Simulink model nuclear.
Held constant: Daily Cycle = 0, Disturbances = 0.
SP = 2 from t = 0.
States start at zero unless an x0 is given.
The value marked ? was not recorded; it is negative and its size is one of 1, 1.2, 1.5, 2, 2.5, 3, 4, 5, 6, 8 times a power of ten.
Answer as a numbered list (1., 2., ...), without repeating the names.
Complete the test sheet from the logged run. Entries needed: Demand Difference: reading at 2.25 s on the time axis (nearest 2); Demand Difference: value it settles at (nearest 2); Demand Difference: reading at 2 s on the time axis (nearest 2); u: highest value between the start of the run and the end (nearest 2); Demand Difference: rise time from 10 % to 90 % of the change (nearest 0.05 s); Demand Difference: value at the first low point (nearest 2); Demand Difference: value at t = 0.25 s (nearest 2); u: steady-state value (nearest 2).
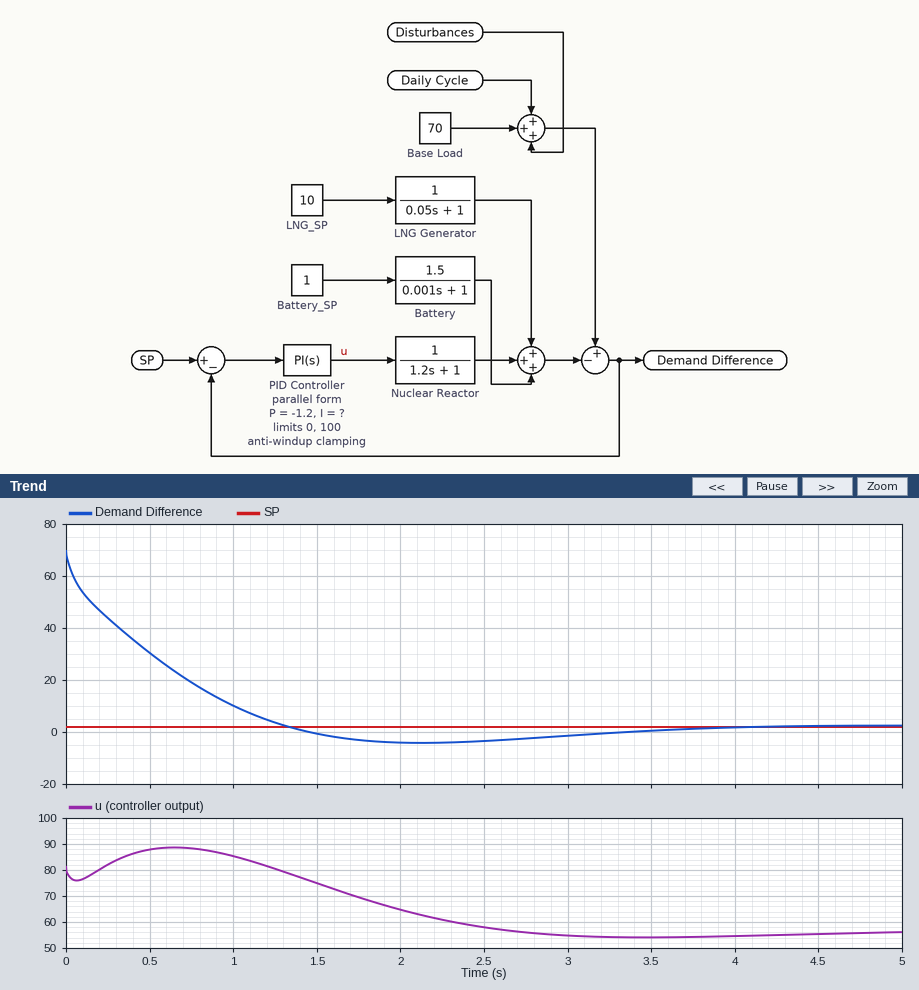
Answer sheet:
1. -4
2. 2
3. -4
4. 88
5. 1.00 s
6. -4
7. 44
8. 56
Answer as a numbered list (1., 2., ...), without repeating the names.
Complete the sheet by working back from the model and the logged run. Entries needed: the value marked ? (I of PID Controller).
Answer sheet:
1. -2.5
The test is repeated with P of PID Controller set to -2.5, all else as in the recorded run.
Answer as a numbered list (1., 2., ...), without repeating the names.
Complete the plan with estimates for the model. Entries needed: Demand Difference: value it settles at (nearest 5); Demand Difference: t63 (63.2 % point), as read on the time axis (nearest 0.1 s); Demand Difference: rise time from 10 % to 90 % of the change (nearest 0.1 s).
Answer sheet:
1. 0
2. 0.5 s
3. 1.2 s
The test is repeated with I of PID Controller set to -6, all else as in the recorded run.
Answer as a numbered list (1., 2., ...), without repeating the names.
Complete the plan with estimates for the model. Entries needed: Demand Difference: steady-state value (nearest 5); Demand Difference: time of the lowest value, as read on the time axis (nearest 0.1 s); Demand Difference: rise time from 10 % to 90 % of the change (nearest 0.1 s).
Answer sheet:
1. 0
2. 1.6 s
3. 0.8 s
